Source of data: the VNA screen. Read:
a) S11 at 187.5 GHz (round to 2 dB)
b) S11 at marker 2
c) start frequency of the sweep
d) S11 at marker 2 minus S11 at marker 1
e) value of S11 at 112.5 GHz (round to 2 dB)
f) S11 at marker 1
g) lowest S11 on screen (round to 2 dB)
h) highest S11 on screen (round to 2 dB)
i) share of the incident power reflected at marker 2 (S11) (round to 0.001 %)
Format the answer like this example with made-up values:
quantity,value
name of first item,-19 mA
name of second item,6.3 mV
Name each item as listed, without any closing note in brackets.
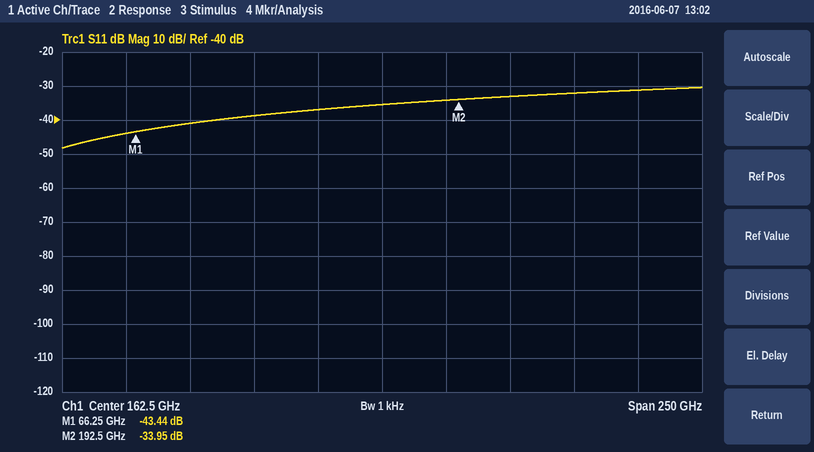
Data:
quantity,value
S11 at 187.5 GHz,-34 dB
S11 at marker 2,-33.95 dB
start frequency of the sweep,37.5 GHz
S11 at marker 2 minus S11 at marker 1,9.49 dB
value of S11 at 112.5 GHz,-38 dB
S11 at marker 1,-43.44 dB
lowest S11 on screen,-48 dB
highest S11 on screen,-30 dB
share of the incident power reflected at marker 2 (S11),0.040 %
